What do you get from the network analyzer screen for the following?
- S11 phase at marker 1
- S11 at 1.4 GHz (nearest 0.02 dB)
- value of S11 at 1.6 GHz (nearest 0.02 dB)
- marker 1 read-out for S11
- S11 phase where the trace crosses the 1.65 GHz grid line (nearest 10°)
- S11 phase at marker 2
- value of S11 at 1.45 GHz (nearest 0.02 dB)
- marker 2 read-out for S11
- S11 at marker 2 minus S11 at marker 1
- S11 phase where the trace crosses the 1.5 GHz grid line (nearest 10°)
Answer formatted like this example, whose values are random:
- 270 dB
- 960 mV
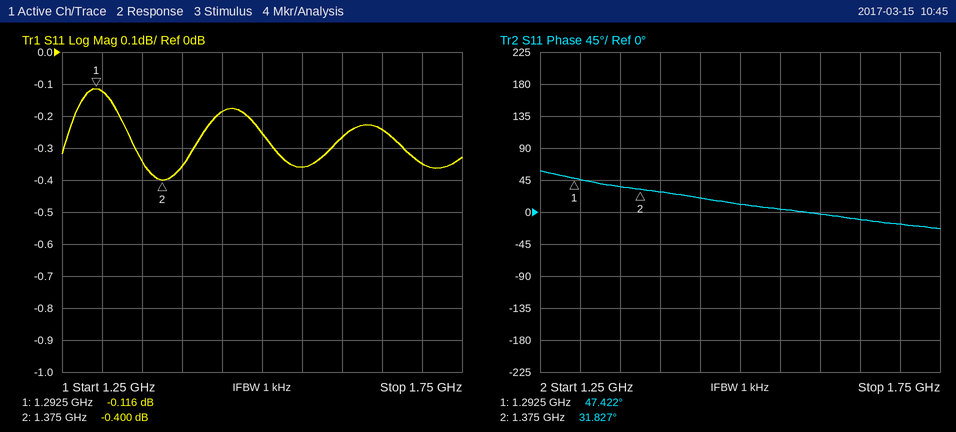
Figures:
- 47.422°
- -0.36 dB
- -0.26 dB
- -0.116 dB
- -10°
- 31.827°
- -0.18 dB
- -0.400 dB
- -0.284 dB
- 10°
